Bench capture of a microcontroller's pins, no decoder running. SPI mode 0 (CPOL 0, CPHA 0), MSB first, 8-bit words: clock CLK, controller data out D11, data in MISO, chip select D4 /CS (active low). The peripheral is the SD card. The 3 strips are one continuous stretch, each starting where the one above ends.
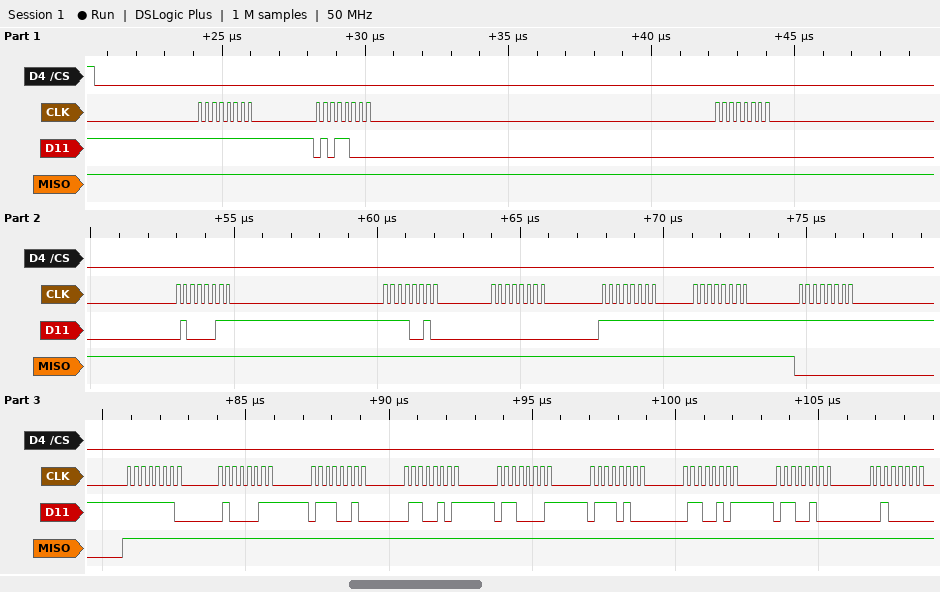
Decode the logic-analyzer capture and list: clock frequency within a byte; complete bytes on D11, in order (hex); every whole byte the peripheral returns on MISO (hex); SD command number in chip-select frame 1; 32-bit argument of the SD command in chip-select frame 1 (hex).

4 MHz
0xFF 0x58 0x00 0x43 0xF2 0x00 0xFF 0xFF 0xFF 0xFE 0x43 0x72 0x65 0x61 0x74 0x65 0x64 0x20
0xFF 0xFF 0xFF 0xFF 0xFF 0xFF 0xFF 0xFF 0x00 0xFF 0xFF 0xFF 0xFF 0xFF 0xFF 0xFF 0xFF 0xFF
CMD24
0x0043F200
